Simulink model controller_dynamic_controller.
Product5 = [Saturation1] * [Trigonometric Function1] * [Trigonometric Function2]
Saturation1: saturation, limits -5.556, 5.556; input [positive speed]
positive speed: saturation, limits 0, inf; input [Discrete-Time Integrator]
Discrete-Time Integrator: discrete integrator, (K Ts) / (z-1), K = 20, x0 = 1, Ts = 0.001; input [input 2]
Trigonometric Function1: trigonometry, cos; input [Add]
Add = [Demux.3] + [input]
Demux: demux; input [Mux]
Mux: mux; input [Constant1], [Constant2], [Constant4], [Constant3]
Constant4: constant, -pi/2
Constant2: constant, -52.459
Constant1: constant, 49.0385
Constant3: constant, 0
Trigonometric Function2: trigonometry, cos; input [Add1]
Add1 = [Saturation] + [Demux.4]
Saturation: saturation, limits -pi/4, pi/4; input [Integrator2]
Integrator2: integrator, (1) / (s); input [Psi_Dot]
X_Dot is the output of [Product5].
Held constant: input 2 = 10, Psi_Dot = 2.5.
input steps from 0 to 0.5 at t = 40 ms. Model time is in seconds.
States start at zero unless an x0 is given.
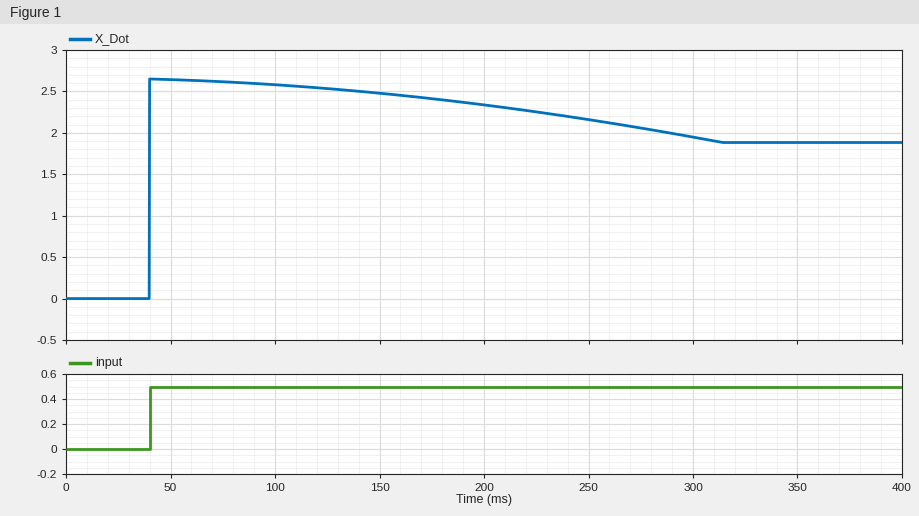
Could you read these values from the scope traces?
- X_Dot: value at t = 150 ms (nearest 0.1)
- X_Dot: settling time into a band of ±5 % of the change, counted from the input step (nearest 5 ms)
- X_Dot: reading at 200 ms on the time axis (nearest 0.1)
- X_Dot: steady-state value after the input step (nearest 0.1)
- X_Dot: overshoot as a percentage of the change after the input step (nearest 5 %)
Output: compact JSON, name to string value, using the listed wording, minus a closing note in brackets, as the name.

{"X_Dot: value at t = 150 ms": "2.5", "X_Dot: settling time into a band of ±5 % of the change, counted from the input step": "255 ms", "X_Dot: reading at 200 ms on the time axis": "2.3", "X_Dot: steady-state value after the input step": "1.9", "X_Dot: overshoot as a percentage of the change after the input step": "40 %"}
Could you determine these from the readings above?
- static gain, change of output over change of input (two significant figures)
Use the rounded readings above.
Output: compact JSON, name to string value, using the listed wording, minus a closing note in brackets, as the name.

{"static gain, change of output over change of input": "3.8"}
